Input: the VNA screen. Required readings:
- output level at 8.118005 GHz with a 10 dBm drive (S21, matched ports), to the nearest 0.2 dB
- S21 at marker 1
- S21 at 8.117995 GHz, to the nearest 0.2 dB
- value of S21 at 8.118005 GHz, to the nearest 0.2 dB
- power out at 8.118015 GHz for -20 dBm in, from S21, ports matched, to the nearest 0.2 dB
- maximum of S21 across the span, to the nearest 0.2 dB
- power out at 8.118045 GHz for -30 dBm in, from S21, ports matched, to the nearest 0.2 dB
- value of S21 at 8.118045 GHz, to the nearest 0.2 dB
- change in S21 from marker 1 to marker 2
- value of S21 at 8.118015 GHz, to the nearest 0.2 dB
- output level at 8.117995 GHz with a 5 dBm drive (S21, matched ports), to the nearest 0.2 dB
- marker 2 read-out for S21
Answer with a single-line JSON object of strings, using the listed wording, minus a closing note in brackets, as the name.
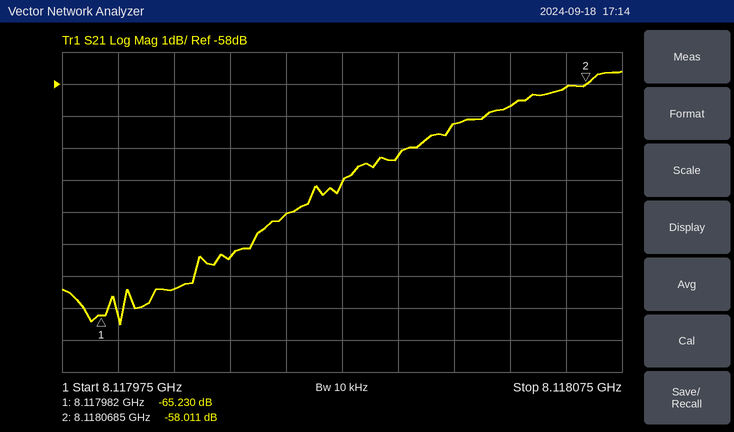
{"output level at 8.118005 GHz with a 10 dBm drive (S21, matched ports), to the nearest 0.2 dB": "-53.4 dBm", "S21 at marker 1": "-65.230 dB", "S21 at 8.117995 GHz, to the nearest 0.2 dB": "-64.4 dB", "value of S21 at 8.118005 GHz, to the nearest 0.2 dB": "-63.4 dB", "power out at 8.118015 GHz for -20 dBm in, from S21, ports matched, to the nearest 0.2 dB": "-82.0 dBm", "maximum of S21 across the span, to the nearest 0.2 dB": "-57.6 dB", "power out at 8.118045 GHz for -30 dBm in, from S21, ports matched, to the nearest 0.2 dB": "-89.2 dBm", "value of S21 at 8.118045 GHz, to the nearest 0.2 dB": "-59.2 dB", "change in S21 from marker 1 to marker 2": "7.219 dB", "value of S21 at 8.118015 GHz, to the nearest 0.2 dB": "-62.0 dB", "output level at 8.117995 GHz with a 5 dBm drive (S21, matched ports), to the nearest 0.2 dB": "-59.4 dBm", "marker 2 read-out for S21": "-58.011 dB"}
